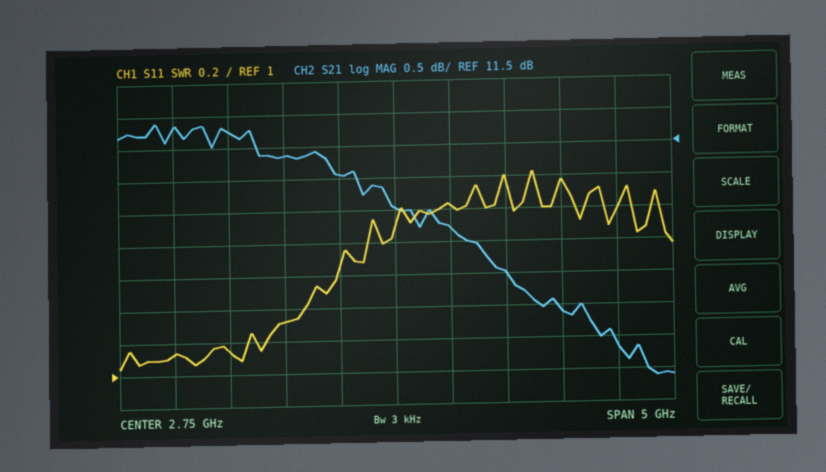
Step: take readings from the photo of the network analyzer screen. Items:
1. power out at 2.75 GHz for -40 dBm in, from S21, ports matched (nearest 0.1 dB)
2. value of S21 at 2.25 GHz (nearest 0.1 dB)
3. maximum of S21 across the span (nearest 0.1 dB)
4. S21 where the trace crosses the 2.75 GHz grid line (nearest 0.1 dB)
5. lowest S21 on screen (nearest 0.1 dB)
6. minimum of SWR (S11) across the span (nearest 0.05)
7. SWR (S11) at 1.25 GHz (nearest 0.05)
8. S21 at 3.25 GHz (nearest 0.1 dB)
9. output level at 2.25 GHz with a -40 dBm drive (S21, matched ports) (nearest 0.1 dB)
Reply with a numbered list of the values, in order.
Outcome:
1. -29.5 dBm
2. 11.1 dB
3. 11.9 dB
4. 10.5 dB
5. 7.9 dB
6. 1.05
7. 1.15
8. 10.2 dB
9. -28.9 dBm
